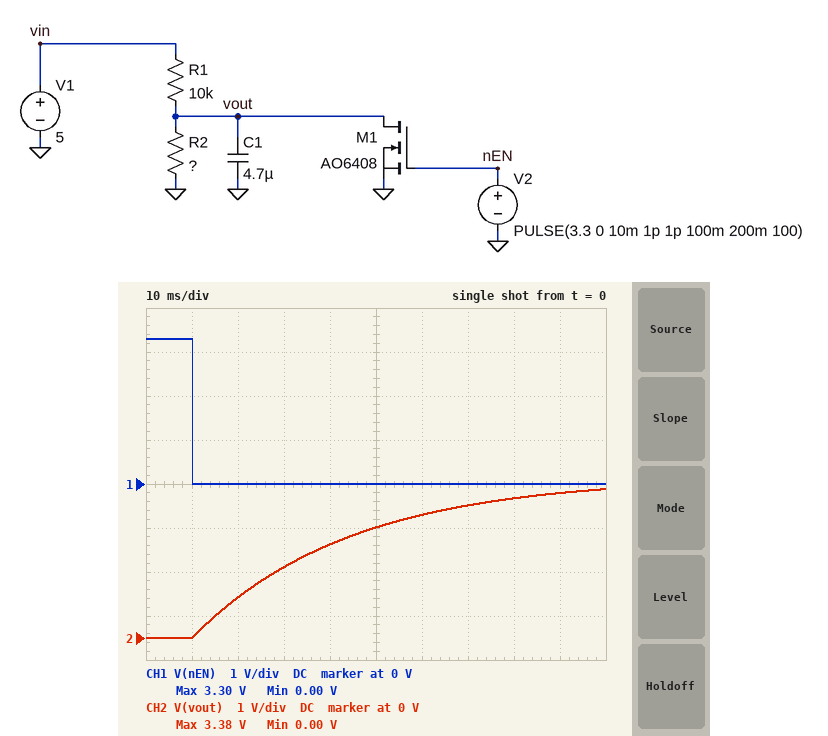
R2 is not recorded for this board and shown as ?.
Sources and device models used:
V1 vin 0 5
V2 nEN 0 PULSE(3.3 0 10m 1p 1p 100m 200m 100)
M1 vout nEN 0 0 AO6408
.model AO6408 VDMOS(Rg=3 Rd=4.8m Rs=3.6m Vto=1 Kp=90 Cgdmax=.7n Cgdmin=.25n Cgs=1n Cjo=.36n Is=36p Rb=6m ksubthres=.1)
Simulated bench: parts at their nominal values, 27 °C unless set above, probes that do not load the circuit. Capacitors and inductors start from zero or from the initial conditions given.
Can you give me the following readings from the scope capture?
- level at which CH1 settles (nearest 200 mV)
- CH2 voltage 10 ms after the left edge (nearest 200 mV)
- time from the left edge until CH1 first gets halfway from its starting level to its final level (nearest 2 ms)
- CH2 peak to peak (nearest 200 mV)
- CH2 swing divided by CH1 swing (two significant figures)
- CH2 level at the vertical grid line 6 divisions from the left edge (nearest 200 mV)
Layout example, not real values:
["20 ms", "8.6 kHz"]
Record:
["0 V", "0 V", "10 ms", "3.4 V", "1.0", "2.8 V"]
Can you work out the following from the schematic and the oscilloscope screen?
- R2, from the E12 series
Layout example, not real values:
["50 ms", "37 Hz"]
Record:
["27 kΩ"]
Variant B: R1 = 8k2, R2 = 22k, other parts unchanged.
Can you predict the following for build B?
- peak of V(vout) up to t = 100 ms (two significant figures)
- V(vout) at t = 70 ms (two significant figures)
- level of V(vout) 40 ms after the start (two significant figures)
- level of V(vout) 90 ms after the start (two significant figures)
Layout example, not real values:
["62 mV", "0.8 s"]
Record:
["3.5 V", "3.2 V", "2.4 V", "3.4 V"]
